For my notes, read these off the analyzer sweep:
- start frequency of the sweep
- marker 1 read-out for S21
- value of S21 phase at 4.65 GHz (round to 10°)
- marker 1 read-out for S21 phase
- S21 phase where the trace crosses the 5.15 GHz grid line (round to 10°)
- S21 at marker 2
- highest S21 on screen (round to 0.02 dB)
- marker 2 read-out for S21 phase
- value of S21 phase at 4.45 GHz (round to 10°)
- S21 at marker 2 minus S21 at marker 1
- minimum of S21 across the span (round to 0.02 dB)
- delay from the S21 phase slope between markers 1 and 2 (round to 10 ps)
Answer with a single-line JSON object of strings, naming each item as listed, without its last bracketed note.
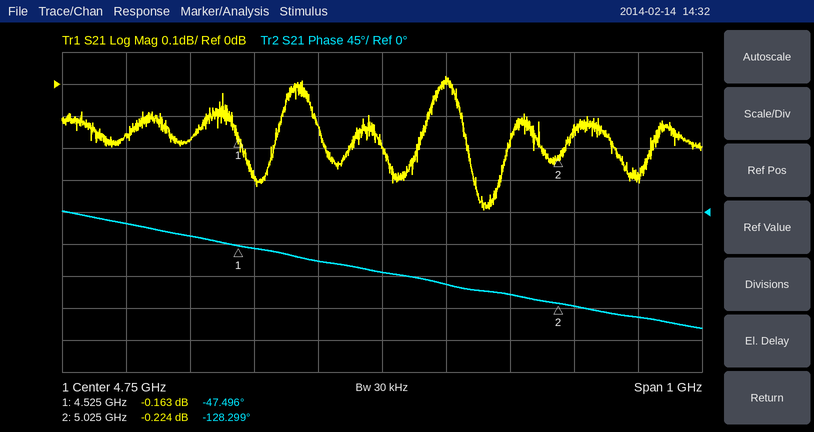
{"start frequency of the sweep": "4.25 GHz", "marker 1 read-out for S21": "-0.163 dB", "value of S21 phase at 4.65 GHz": "-70°", "marker 1 read-out for S21 phase": "-47.496°", "S21 phase where the trace crosses the 5.15 GHz grid line": "-150°", "S21 at marker 2": "-0.224 dB", "highest S21 on screen": "0.02 dB", "marker 2 read-out for S21 phase": "-128.299°", "value of S21 phase at 4.45 GHz": "-30°", "S21 at marker 2 minus S21 at marker 1": "-0.061 dB", "minimum of S21 across the span": "-0.40 dB", "delay from the S21 phase slope between markers 1 and 2": "450 ps"}
